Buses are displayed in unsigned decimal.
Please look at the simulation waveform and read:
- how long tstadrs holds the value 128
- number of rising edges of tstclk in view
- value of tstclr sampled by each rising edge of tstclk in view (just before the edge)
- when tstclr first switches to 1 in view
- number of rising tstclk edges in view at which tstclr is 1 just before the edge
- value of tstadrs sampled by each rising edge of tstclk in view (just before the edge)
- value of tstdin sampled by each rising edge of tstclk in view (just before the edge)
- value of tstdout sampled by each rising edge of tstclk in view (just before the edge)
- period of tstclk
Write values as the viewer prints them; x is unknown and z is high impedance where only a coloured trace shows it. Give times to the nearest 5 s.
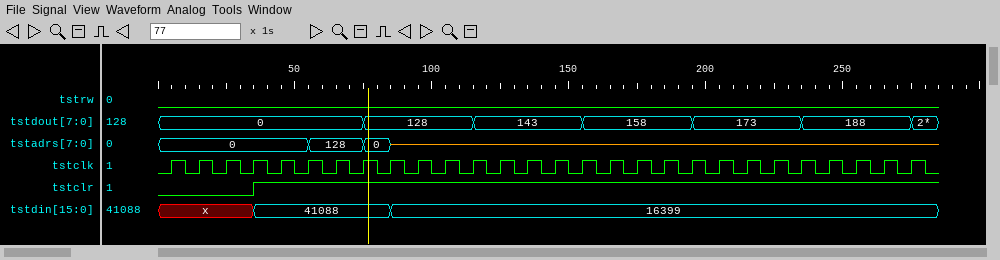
20 s
28
0 0 0 0 1 1 1 1 1 1 1 1 1 1 1 1 1 1 1 1 1 1 1 1 1 1 1 1
35 s
24
0, 0, 0, 0, 0, 0, 128, 128, 0, z, z, z, z, z, z, z, z, z, z, z, z, z, z, z, z, z, z, z
x, x, x, x, 41088, 41088, 41088, 41088, 41088, 16399, 16399, 16399, 16399, 16399, 16399, 16399, 16399, 16399, 16399, 16399, 16399, 16399, 16399, 16399, 16399, 16399, 16399, 16399
0, 0, 0, 0, 0, 0, 0, 0, 128, 128, 128, 128, 143, 143, 143, 143, 158, 158, 158, 158, 173, 173, 173, 173, 188, 188, 188, 188
10 s
